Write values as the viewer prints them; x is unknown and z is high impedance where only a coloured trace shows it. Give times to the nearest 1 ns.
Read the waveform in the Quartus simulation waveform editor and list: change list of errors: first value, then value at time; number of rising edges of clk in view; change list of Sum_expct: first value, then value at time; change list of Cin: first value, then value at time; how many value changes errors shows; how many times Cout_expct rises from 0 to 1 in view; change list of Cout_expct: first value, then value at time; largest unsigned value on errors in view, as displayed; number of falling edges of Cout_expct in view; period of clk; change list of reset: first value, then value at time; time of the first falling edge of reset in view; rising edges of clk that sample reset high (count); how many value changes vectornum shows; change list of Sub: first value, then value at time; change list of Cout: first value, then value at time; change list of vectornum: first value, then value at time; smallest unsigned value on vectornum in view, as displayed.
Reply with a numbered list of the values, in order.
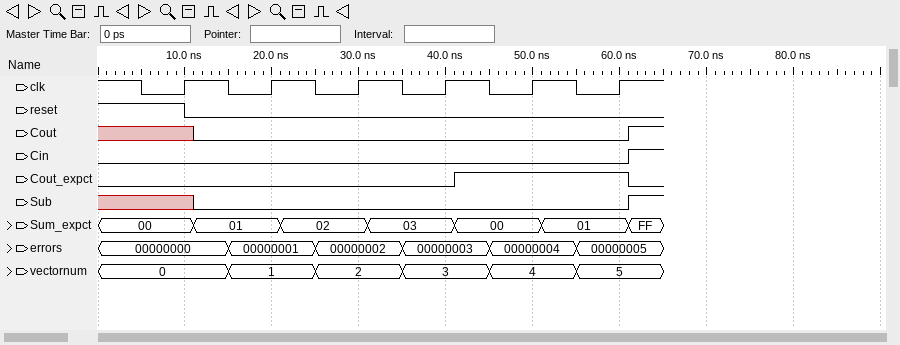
1. 00000000, 00000001 at 15 ns, 00000002 at 25 ns, 00000003 at 35 ns, 00000004 at 45 ns, 00000005 at 55 ns
2. 6
3. 00, 01 at 11 ns, 02 at 21 ns, 03 at 31 ns, 00 at 41 ns, 01 at 51 ns, FF at 61 ns
4. 0, 1 at 61 ns
5. 5
6. 1
7. 0, 1 at 41 ns, 0 at 61 ns
8. 00000005
9. 1
10. 10 ns
11. 1, 0 at 10 ns
12. 10 ns
13. 1
14. 5
15. x, 0 at 11 ns, 1 at 61 ns
16. x, 0 at 11 ns, 1 at 61 ns
17. 0, 1 at 15 ns, 2 at 25 ns, 3 at 35 ns, 4 at 45 ns, 5 at 55 ns
18. 0
